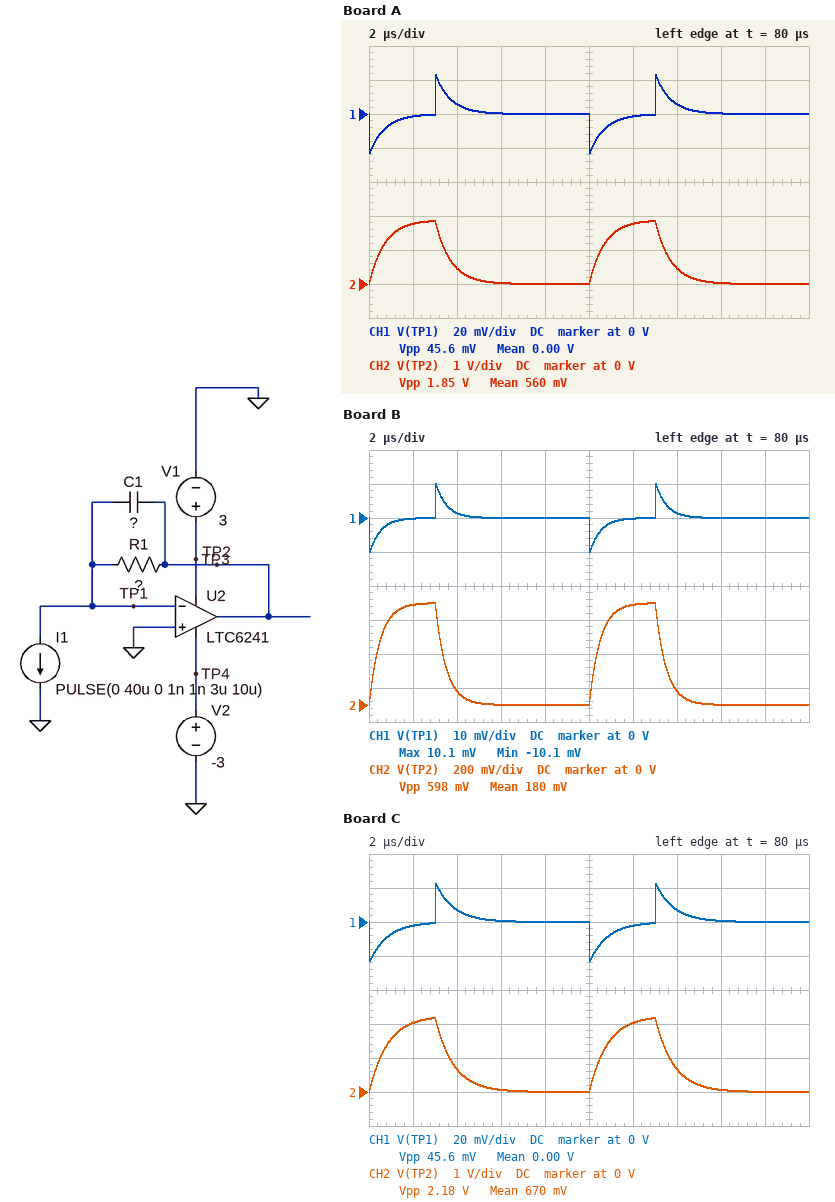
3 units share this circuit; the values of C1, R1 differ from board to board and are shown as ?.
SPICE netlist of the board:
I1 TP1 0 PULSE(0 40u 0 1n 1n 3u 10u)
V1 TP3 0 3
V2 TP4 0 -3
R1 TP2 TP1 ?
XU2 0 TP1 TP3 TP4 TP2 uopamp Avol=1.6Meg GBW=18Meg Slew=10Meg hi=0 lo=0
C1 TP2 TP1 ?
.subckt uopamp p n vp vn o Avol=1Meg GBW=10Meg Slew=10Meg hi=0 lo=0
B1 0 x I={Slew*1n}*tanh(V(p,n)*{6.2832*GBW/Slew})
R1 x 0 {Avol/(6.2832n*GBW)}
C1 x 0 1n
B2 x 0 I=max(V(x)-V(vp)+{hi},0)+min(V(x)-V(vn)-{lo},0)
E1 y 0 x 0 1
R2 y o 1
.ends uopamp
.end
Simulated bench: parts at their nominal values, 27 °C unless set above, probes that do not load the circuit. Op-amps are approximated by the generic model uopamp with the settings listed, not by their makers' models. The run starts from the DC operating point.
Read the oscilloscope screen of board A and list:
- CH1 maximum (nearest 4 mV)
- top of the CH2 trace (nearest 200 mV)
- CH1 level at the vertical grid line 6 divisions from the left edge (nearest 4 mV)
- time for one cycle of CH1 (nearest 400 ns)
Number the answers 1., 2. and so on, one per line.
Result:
1. 24 mV
2. 1.8 V
3. 0 V
4. 10.0 µs
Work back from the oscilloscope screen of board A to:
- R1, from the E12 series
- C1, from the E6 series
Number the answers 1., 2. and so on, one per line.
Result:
1. 47 kΩ
2. 15 pF
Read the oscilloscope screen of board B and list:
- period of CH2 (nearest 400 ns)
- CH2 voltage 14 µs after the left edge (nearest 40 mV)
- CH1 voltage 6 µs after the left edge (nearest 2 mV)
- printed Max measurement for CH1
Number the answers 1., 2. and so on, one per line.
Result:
1. 10.0 µs
2. 80 mV
3. 0 V
4. 10.1 mV
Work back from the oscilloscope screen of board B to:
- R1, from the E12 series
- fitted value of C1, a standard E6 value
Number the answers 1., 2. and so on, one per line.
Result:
1. 15 kΩ
2. 33 pF
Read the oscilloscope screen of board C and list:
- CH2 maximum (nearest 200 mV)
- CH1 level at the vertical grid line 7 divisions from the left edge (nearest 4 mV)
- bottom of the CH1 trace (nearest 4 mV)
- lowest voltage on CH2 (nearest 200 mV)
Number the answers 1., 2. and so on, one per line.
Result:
1. 2.2 V
2. 8 mV
3. -24 mV
4. 0 V
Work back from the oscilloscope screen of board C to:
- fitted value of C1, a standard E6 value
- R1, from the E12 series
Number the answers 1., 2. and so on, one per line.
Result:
1. 15 pF
2. 56 kΩ
